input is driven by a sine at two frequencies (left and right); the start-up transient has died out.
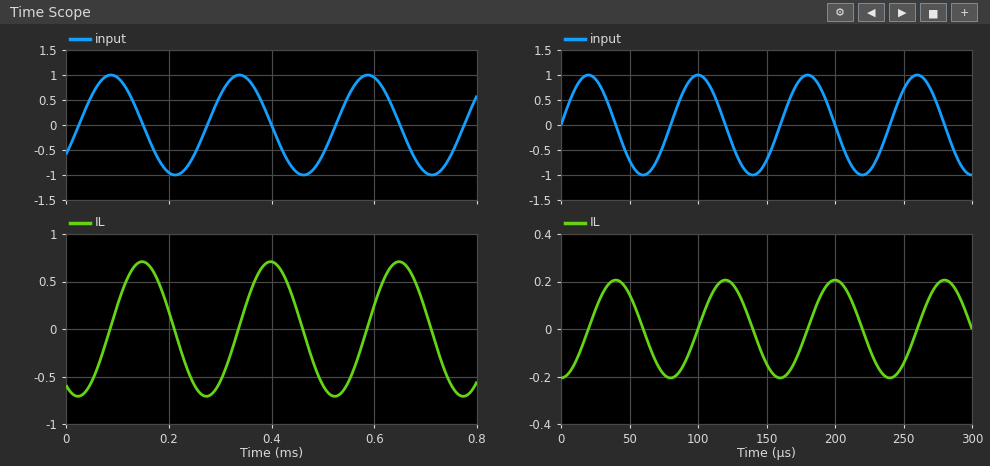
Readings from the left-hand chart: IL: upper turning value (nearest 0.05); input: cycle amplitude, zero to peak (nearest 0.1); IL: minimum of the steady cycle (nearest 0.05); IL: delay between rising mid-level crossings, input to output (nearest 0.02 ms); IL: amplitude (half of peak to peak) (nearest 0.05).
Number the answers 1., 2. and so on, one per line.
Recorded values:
1. 0.70
2. 1.0
3. -0.70
4. 0.06 ms
5. 0.70
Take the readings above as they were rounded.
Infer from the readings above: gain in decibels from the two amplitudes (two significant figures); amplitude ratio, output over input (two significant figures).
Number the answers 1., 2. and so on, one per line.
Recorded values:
1. -3.1 dB
2. 0.70
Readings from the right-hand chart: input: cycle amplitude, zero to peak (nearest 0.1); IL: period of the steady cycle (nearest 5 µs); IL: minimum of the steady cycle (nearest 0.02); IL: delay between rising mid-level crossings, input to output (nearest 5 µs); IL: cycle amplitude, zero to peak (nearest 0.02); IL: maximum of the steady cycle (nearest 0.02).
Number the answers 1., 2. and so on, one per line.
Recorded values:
1. 1.0
2. 80 µs
3. -0.20
4. 20 µs
5. 0.20
6. 0.20
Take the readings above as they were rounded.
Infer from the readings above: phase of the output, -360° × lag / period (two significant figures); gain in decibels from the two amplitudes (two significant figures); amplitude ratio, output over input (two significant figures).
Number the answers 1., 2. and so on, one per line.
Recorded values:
1. -90°
2. -14 dB
3. 0.20
